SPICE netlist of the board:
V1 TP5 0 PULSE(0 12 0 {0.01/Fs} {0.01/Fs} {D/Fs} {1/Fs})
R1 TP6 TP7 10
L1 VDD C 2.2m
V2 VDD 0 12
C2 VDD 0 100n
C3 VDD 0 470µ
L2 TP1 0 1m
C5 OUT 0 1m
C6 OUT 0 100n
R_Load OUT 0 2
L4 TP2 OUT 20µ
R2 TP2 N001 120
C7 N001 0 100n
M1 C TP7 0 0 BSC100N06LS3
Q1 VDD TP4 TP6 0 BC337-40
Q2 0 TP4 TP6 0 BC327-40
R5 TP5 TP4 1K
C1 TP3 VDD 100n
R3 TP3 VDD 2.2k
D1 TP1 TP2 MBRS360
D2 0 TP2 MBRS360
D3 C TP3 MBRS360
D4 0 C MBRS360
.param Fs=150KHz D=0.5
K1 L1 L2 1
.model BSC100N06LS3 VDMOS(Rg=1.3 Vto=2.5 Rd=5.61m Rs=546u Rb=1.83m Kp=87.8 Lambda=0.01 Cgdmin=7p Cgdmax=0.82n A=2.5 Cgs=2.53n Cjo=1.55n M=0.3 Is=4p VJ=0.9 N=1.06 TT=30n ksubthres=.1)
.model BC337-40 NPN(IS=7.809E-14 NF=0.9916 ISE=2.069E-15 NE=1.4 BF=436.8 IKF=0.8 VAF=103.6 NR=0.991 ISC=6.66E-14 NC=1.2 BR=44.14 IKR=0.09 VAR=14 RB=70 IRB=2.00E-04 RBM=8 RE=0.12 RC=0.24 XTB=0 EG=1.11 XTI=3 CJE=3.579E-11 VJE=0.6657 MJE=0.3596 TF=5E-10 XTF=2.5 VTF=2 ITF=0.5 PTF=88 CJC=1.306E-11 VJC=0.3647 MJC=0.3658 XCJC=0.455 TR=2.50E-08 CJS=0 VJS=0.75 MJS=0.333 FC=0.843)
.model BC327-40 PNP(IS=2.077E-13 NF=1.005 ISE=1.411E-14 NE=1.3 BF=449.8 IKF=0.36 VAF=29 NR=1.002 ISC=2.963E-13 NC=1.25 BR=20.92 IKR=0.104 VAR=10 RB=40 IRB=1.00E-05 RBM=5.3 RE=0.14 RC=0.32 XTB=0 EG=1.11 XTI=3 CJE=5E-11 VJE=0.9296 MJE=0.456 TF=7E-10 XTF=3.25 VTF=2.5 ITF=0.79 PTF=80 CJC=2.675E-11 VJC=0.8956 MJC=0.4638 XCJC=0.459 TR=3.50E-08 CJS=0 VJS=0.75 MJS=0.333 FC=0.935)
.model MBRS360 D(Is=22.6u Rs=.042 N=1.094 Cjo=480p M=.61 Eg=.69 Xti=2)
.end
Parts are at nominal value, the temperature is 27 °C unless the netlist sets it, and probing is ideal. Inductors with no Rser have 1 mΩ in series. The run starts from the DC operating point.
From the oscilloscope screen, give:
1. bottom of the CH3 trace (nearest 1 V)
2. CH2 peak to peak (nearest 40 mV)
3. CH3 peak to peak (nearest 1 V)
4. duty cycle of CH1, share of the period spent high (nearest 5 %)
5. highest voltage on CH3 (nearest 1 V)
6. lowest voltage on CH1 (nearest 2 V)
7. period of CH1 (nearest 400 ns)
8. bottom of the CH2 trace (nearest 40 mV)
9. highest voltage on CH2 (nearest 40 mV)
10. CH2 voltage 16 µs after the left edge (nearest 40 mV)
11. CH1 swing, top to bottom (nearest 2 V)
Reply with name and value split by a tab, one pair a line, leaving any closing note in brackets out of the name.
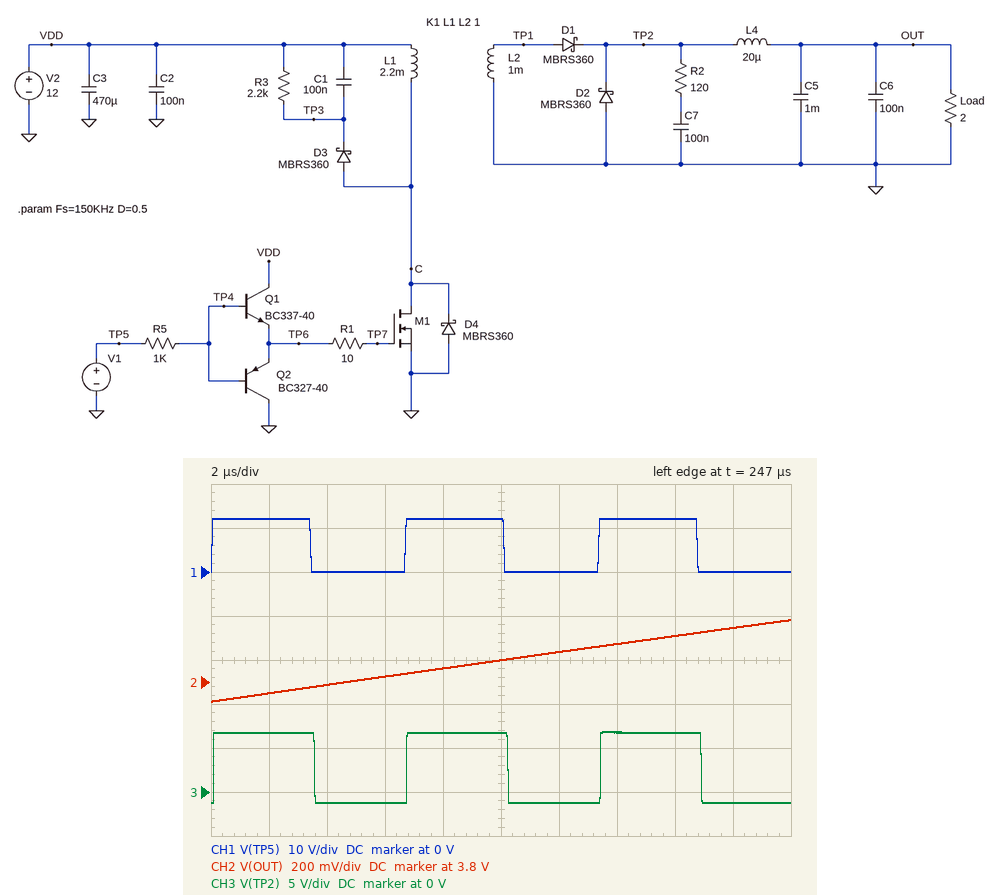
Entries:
bottom of the CH3 trace	-1 V
CH2 peak to peak	360 mV
CH3 peak to peak	8 V
duty cycle of CH1, share of the period spent high	50 %
highest voltage on CH3	7 V
lowest voltage on CH1	0 V
period of CH1	6.8 µs
bottom of the CH2 trace	3.72 V
highest voltage on CH2	4.08 V
CH2 voltage 16 µs after the left edge	4.00 V
CH1 swing, top to bottom	12 V
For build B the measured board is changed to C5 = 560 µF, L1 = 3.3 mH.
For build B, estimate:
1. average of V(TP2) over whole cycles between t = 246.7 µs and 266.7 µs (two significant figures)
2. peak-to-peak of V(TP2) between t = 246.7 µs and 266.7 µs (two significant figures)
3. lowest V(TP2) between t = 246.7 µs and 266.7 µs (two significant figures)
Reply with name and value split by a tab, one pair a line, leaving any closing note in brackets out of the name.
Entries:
average of V(TP2) over whole cycles between t = 246.7 µs and 266.7 µs	2.7 V
peak-to-peak of V(TP2) between t = 246.7 µs and 266.7 µs	6.6 V
lowest V(TP2) between t = 246.7 µs and 266.7 µs	-790 mV
